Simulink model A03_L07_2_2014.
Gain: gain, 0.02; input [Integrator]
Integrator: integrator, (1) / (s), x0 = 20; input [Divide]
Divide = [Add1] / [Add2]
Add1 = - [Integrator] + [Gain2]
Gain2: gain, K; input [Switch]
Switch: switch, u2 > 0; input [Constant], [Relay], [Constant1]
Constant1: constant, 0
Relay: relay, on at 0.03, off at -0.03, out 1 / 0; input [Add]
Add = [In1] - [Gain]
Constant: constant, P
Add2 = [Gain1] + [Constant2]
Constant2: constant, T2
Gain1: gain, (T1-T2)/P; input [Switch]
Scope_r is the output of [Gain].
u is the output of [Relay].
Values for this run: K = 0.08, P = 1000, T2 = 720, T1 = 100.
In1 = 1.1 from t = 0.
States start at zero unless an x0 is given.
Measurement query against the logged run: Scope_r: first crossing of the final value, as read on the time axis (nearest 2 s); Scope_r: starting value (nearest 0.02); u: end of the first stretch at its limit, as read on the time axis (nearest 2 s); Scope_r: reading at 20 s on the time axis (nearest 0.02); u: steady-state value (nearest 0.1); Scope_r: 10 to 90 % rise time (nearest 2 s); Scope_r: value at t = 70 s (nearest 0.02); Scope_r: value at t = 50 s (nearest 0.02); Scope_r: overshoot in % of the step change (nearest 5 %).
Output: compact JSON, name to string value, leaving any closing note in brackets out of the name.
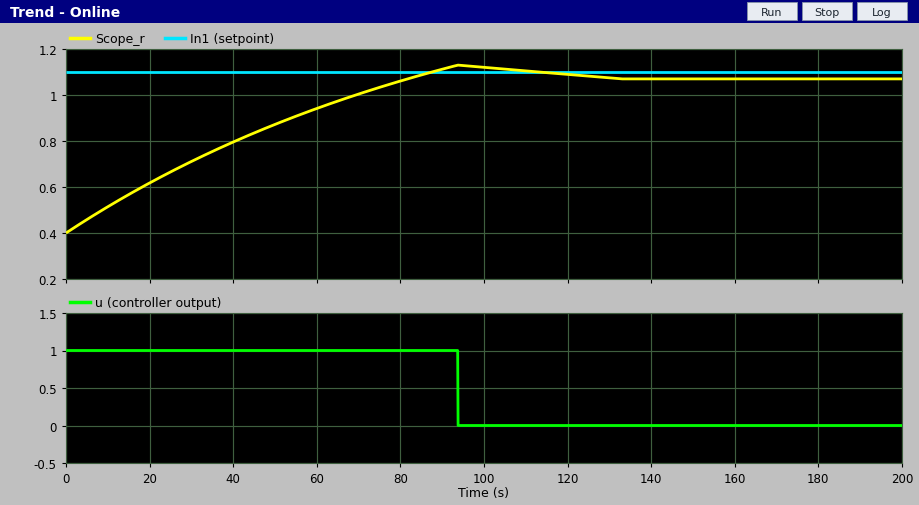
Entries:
{"Scope_r: first crossing of the final value, as read on the time axis": "82 s", "Scope_r: starting value": "0.40", "u: end of the first stretch at its limit, as read on the time axis": "94 s", "Scope_r: reading at 20 s on the time axis": "0.62", "u: steady-state value": "0.0", "Scope_r: 10 to 90 % rise time": "64 s", "Scope_r: value at t = 70 s": "1.00", "Scope_r: value at t = 50 s": "0.88", "Scope_r: overshoot in % of the step change": "10 %"}
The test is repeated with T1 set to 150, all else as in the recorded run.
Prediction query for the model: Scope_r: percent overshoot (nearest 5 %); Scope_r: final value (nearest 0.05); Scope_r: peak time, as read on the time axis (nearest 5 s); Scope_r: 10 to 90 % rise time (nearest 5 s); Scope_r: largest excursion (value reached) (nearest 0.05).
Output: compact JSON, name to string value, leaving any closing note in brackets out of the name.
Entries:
{"Scope_r: percent overshoot": "10 %", "Scope_r: final value": "1.05", "Scope_r: peak time, as read on the time axis": "140 s", "Scope_r: 10 to 90 % rise time": "95 s", "Scope_r: largest excursion (value reached)": "1.15"}
